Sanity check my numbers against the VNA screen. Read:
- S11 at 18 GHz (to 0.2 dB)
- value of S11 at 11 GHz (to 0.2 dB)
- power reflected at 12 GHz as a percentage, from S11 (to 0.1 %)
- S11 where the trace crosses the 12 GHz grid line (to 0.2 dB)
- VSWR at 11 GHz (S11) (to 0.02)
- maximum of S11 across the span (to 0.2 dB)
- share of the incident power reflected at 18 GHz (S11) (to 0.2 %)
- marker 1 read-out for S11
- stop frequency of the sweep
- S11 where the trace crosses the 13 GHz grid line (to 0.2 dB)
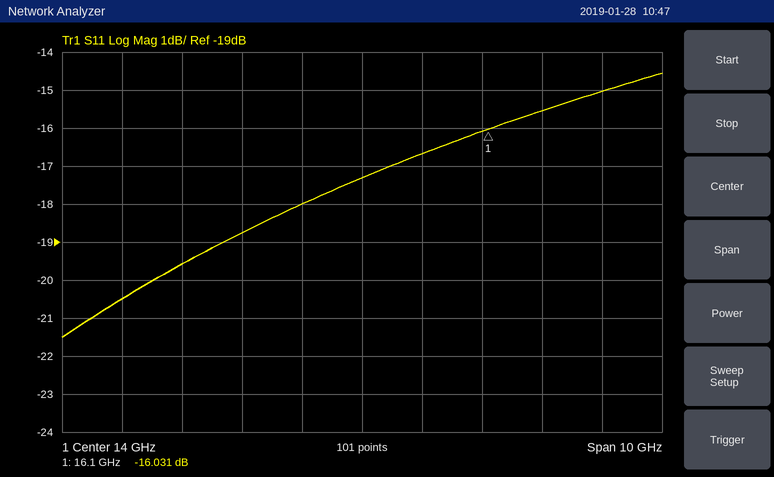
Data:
-15.0 dB
-19.6 dB
1.3 %
-18.8 dB
1.24
-14.6 dB
3.2 %
-16.031 dB
19 GHz
-18.0 dB
